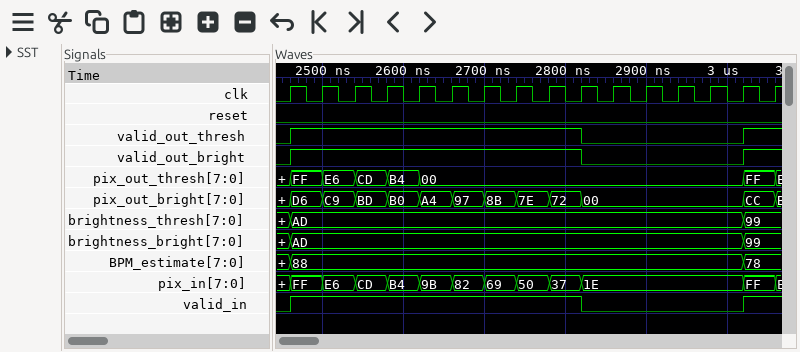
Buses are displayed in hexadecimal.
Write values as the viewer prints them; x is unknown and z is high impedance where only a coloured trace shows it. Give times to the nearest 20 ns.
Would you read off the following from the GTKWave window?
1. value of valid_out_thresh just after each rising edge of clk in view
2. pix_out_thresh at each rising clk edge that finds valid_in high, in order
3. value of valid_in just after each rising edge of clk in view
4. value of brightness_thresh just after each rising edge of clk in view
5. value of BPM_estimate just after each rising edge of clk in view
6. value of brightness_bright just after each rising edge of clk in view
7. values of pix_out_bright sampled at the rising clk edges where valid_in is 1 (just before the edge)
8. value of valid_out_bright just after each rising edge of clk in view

1 1 1 1 1 1 1 1 1 0 0 0 0 0 1 1
FF, E6, CD, B4, 00, 00, 00, 00, 00, FF
1 1 1 1 1 1 1 1 1 0 0 0 0 0 1 1
AD, AD, AD, AD, AD, AD, AD, AD, AD, AD, AD, AD, AD, AD, 99, 99
88, 88, 88, 88, 88, 88, 88, 88, 88, 88, 88, 88, 88, 88, 78, 78
AD, AD, AD, AD, AD, AD, AD, AD, AD, AD, AD, AD, AD, AD, 99, 99
D6, C9, BD, B0, A4, 97, 8B, 7E, 72, CC
1 1 1 1 1 1 1 1 1 0 0 0 0 0 1 1
